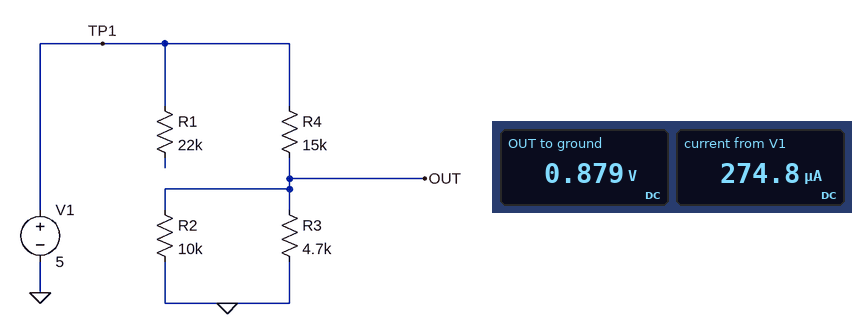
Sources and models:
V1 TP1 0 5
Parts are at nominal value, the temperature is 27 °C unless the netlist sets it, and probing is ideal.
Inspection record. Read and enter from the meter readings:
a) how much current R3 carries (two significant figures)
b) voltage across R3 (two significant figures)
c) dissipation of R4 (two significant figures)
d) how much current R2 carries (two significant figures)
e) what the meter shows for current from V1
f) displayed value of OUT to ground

190 µA
880 mV
1.1 mW
88 µA
274.8 µA
0.879 V
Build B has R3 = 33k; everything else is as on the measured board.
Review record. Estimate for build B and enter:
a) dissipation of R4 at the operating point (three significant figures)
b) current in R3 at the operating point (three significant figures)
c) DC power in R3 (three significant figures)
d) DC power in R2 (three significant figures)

729 µW
51.3 µA
86.8 µW
286 µW
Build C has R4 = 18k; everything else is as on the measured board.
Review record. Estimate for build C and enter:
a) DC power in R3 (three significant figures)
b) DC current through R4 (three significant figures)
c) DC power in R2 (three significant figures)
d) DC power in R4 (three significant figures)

121 µW
236 µA
56.9 µW
1.00 mW
